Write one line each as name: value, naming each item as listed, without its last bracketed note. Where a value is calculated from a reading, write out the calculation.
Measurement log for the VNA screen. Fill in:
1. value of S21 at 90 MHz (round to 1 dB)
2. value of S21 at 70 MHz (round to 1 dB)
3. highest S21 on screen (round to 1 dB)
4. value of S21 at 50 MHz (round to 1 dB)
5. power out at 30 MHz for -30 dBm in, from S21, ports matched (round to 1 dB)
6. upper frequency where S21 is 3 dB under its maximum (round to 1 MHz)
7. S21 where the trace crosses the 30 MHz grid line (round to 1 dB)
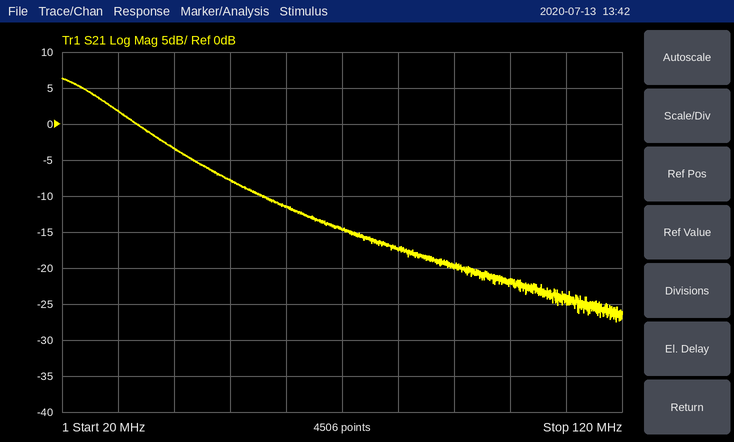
value of S21 at 90 MHz: -20 dB
value of S21 at 70 MHz: -15 dB
highest S21 on screen: 6 dB
value of S21 at 50 MHz: -8 dB
power out at 30 MHz for -30 dBm in, from S21, ports matched: -30 dBm + (2 dB) = -28 dBm
upper frequency where S21 is 3 dB under its maximum: 27 MHz
S21 where the trace crosses the 30 MHz grid line: 2 dB
